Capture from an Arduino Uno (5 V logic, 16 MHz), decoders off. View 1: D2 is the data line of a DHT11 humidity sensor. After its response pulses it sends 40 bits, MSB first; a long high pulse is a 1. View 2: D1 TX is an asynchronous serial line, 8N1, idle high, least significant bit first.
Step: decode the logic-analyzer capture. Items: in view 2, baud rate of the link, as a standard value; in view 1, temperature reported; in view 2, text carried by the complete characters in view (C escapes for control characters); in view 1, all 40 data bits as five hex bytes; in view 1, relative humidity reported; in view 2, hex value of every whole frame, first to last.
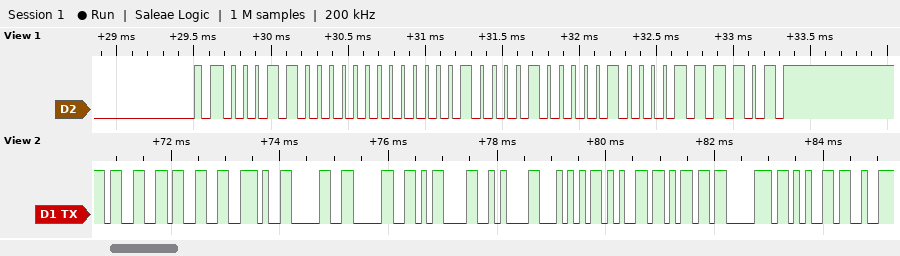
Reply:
9600 baud
33.4 °C
"33.00\r\nTempe"
18 00 21 04 3D
24 %
33 33 2E 30 30 0D 0A 54 65 6D 70 65
